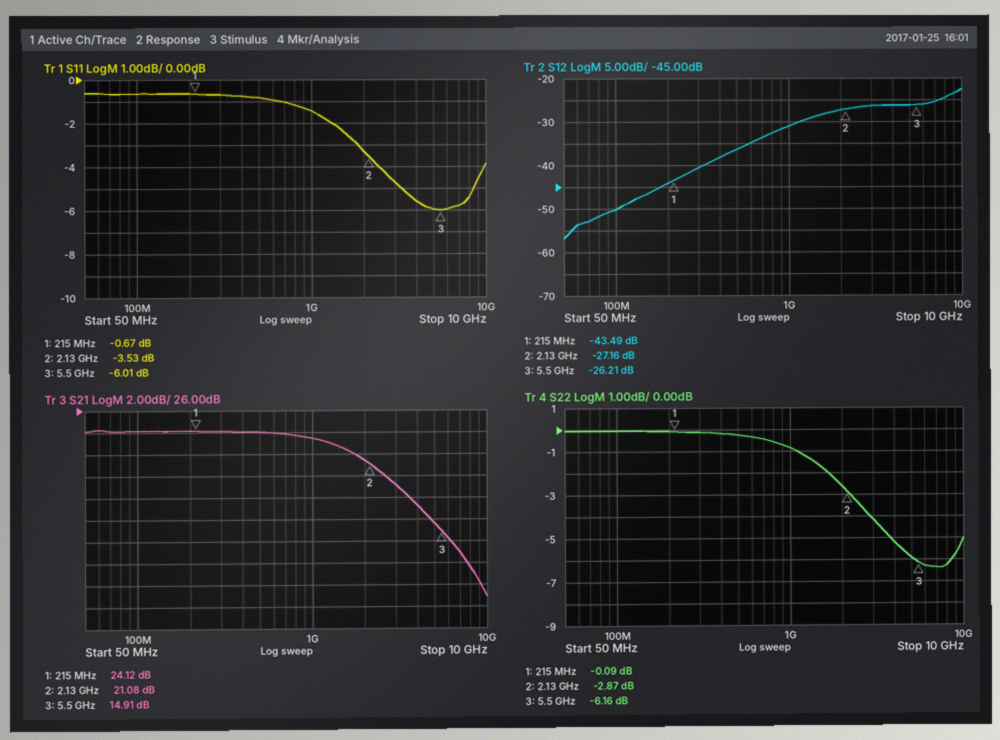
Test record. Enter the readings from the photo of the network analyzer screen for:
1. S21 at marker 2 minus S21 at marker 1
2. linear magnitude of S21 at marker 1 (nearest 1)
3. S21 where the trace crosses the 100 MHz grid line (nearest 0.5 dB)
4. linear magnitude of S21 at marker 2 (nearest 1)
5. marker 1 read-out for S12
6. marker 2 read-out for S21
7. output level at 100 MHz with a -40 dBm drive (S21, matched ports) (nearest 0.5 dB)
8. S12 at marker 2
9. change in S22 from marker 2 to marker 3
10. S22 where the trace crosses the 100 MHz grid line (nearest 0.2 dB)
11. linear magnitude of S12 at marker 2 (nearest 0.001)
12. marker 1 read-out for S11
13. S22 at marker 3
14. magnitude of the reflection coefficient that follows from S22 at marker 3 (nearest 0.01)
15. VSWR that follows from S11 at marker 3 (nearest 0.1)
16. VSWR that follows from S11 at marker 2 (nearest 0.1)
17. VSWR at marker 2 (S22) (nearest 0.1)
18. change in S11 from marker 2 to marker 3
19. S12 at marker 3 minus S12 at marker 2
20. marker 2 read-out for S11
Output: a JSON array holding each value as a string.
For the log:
["-3.04 dB", "16", "24.0 dB", "11", "-43.49 dB", "21.08 dB", "-16.0 dBm", "-27.16 dB", "-3.29 dB", "0.0 dB", "0.044", "-0.67 dB", "-6.16 dB", "0.49", "3.0", "5.0", "6.1", "-2.48 dB", "0.95 dB", "-3.53 dB"]
